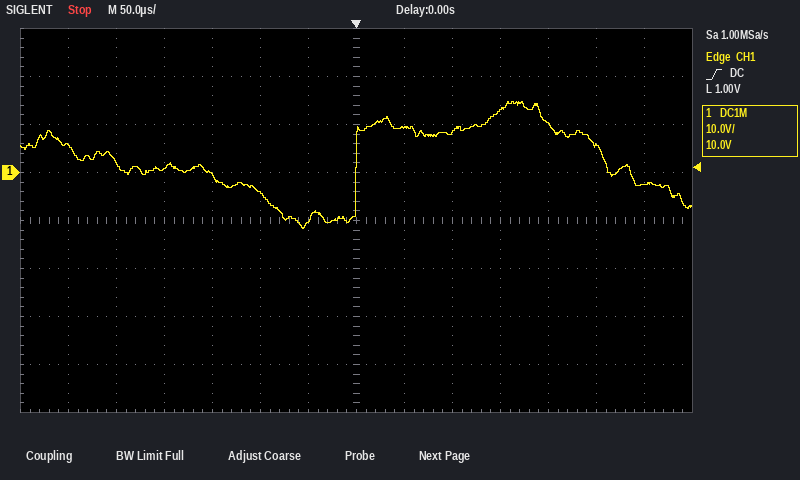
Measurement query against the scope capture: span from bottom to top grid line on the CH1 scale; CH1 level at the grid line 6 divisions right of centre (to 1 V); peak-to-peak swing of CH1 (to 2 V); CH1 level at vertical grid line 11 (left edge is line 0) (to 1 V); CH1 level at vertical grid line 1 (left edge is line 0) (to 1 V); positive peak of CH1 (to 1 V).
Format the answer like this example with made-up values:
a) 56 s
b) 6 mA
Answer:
a) 80 V
b) -2 V
c) 26 V
d) 10 V
e) 6 V
f) 15 V
